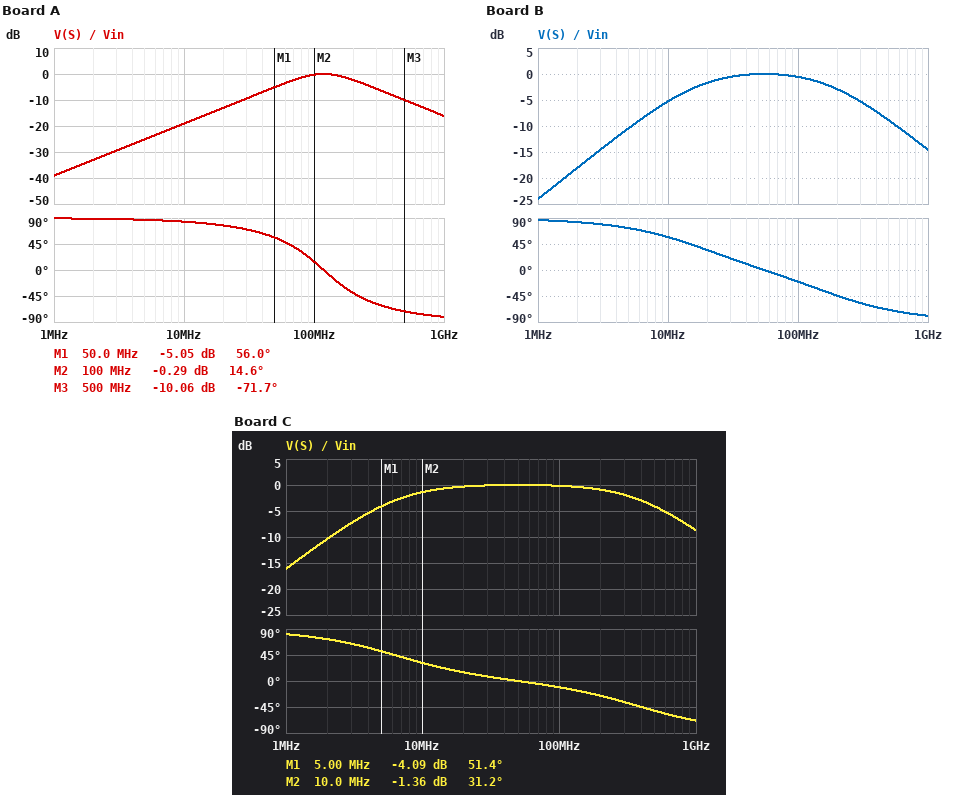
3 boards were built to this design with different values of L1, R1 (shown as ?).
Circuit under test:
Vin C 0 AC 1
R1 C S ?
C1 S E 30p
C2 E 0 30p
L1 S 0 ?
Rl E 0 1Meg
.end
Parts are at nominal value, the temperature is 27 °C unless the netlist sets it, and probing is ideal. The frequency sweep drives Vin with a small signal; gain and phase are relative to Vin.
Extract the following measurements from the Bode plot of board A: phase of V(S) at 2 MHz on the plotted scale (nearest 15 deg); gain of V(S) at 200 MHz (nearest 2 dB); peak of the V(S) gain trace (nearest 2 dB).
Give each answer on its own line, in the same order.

90 deg
-2 dB
0 dB
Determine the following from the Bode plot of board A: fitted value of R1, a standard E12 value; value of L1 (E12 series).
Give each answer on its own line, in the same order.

68 Ω
120 nH
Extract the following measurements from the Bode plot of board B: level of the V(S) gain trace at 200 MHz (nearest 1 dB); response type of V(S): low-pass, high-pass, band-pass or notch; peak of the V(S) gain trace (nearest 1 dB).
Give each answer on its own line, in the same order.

-3 dB
band-pass
0 dB
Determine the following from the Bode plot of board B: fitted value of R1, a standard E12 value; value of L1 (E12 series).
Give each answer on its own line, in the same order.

56 Ω
560 nH
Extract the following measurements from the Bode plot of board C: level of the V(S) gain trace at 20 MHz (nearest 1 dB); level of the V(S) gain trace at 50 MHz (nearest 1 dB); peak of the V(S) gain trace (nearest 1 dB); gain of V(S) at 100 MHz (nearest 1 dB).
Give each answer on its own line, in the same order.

0 dB
0 dB
0 dB
0 dB
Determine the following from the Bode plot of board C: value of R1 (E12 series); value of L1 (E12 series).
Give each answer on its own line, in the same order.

27 Ω
680 nH
